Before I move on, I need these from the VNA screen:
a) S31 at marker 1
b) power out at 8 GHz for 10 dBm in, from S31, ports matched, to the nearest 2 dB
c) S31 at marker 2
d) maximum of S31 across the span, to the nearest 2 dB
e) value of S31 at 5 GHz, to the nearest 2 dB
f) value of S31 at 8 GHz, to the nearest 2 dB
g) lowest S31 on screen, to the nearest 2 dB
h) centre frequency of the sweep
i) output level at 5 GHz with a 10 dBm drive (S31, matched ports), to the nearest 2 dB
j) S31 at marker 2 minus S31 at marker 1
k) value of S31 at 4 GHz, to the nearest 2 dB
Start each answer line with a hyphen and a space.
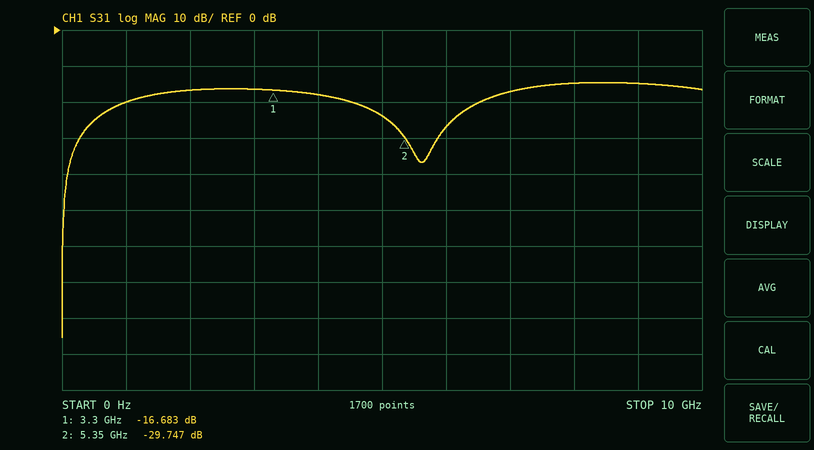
- -16.683 dB
- -4 dBm
- -29.747 dB
- -14 dB
- -24 dB
- -14 dB
- -86 dB
- 5 GHz
- -14 dBm
- -13.064 dB
- -18 dB
